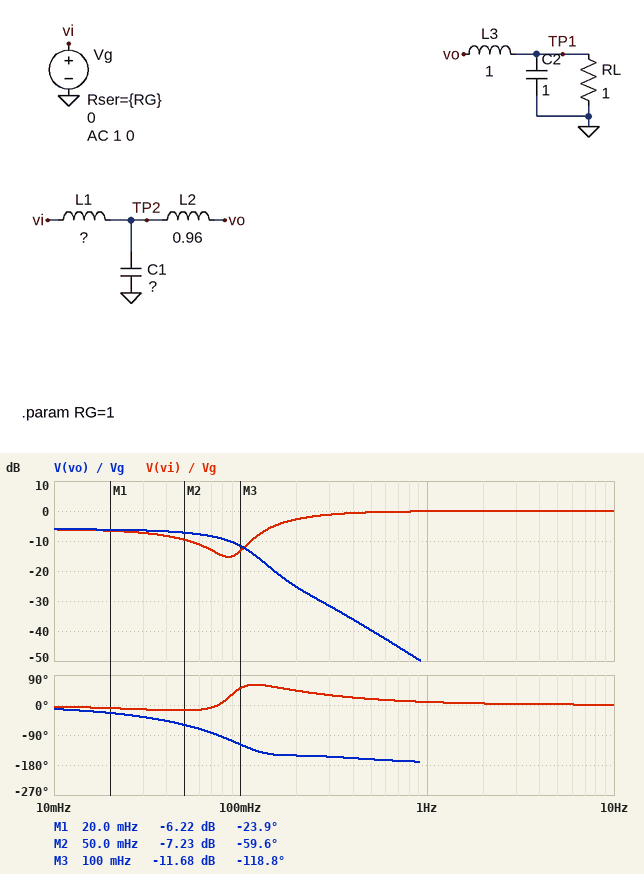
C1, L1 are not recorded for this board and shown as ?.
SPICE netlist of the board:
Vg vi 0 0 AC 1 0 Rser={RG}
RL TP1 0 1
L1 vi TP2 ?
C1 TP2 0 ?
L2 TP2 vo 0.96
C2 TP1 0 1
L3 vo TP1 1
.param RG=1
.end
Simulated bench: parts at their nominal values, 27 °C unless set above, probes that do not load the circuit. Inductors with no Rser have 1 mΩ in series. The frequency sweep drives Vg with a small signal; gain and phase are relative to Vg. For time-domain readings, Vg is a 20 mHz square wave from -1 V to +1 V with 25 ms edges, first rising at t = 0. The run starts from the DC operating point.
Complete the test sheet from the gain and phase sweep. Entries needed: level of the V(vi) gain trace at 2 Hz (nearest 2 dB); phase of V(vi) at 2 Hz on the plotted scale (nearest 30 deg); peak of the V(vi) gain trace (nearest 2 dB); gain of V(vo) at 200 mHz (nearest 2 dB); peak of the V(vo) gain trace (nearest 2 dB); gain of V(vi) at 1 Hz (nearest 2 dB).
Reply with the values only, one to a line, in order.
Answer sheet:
0 dB
0 deg
0 dB
-26 dB
-6 dB
0 dB
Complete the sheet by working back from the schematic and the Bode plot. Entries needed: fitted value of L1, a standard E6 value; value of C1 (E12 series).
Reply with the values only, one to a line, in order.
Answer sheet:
1 H
4.7 F
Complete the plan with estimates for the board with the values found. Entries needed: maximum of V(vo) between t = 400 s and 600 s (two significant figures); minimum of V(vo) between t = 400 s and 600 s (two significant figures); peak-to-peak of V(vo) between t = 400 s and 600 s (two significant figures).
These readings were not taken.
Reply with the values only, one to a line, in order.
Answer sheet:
510 mV
-510 mV
1.0 V
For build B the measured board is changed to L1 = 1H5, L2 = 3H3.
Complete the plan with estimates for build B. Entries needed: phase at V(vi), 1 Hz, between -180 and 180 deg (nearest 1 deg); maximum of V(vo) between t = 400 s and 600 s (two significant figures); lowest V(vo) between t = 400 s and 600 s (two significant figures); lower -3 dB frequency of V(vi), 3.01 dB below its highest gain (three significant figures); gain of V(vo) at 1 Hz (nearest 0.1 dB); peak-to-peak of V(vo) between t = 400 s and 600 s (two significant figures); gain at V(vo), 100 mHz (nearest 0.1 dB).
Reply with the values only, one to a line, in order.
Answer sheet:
6 deg
570 mV
-570 mV
135 mHz
-61.7 dB
1.1 V
-19.5 dB
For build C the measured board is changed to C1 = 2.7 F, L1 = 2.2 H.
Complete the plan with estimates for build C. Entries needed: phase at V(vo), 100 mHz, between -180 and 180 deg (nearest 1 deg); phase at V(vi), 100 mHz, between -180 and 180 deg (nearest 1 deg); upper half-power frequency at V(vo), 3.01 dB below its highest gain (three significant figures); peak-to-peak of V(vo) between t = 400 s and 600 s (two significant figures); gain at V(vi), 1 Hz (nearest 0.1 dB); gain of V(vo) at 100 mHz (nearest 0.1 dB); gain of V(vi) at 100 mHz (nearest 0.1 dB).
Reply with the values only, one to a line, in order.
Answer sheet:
-116 deg
31 deg
103 mHz
1.1 V
0 dB
-8.7 dB
-5.9 dB
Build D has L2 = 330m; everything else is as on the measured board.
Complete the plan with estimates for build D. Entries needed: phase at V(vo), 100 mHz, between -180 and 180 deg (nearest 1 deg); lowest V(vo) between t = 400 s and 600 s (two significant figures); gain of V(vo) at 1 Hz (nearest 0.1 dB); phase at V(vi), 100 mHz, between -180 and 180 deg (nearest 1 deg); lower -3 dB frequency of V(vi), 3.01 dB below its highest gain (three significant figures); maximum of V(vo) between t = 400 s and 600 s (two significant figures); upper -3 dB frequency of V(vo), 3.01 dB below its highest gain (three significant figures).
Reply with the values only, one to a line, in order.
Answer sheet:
-93 deg
-500 mV
-47.9 dB
47 deg
193 mHz
500 mV
75.7 mHz
